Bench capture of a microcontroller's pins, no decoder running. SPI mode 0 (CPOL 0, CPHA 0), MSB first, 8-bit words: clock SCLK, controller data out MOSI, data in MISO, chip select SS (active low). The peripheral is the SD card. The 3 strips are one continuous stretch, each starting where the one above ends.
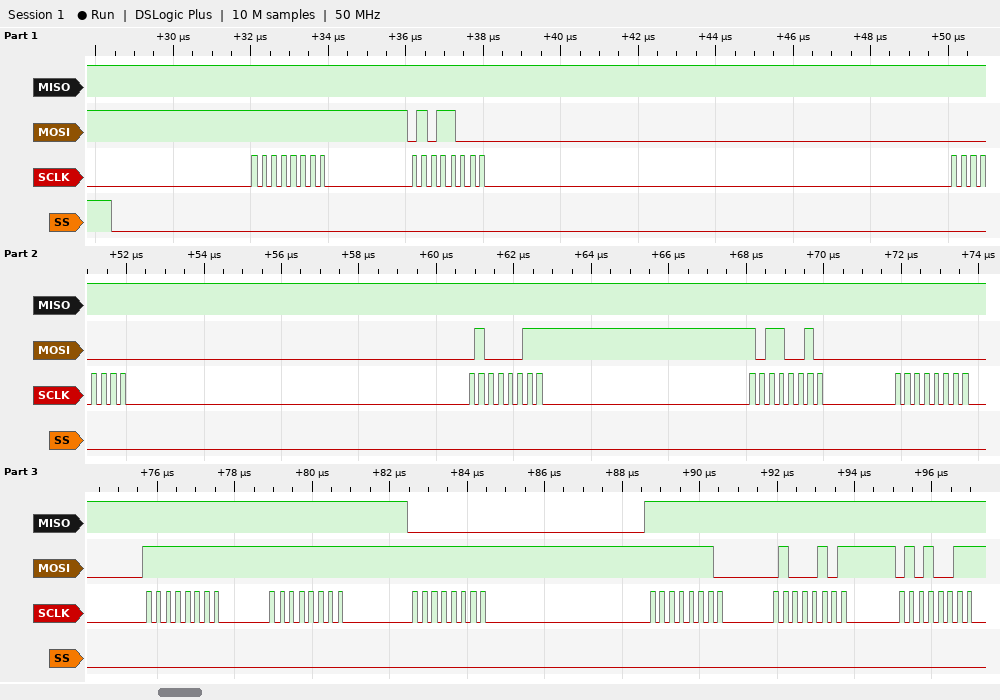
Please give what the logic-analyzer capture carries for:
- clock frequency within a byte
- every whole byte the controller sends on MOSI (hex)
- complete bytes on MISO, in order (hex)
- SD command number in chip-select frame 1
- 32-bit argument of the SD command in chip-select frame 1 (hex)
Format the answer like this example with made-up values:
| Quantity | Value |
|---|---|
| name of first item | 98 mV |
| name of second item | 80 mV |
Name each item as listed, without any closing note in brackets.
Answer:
| Quantity | Value |
|---|---|
| clock frequency within a byte | 4 MHz |
| every whole byte the controller sends on MOSI | 0xFF 0x58 0x00 0x43 0xB2 0x00 0xFF 0xFF 0xFF 0xFE 0x45 0x53 |
| complete bytes on MISO, in order | 0xFF 0xFF 0xFF 0xFF 0xFF 0xFF 0xFF 0xFF 0x00 0xFF 0xFF 0xFF |
| SD command number in chip-select frame 1 | CMD24 |
| 32-bit argument of the SD command in chip-select frame 1 | 0x0043B200 |
